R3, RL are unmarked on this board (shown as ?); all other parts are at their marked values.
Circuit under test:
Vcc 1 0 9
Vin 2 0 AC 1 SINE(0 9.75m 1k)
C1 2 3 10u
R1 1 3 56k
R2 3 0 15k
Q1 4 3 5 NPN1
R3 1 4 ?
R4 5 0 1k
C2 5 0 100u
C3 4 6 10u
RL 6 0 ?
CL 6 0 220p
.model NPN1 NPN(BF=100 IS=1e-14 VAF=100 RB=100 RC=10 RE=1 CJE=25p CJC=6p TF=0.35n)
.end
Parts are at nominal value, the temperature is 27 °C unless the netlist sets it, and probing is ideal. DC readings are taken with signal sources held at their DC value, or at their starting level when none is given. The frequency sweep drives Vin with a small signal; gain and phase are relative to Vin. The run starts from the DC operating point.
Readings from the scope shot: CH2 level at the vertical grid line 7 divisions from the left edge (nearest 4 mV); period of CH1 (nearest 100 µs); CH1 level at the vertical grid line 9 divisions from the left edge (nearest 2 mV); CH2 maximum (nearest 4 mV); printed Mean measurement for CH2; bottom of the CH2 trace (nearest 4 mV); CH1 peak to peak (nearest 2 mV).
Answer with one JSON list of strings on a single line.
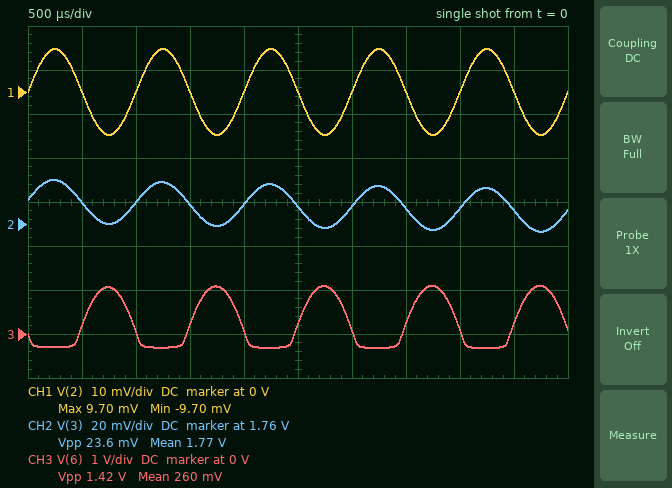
["1.768 V", "1.0 ms", "0 V", "1.780 V", "1.77 V", "1.756 V", "20 mV"]
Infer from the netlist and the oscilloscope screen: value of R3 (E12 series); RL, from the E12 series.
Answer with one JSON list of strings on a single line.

["6.8 kΩ", "5.6 kΩ"]
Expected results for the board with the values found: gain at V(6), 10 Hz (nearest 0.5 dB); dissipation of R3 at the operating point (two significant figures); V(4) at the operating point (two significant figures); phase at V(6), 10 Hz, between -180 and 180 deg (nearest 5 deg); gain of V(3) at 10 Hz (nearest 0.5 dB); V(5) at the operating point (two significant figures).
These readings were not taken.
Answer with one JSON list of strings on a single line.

["24.5 dB", "8.2 mW", "1.5 V", "-90 deg", "-1.0 dB", "1.1 V"]
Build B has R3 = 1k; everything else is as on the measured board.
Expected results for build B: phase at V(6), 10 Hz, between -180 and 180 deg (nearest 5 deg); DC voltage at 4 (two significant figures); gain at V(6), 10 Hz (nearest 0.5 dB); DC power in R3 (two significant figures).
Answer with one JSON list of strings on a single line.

["-85 deg", "7.9 V", "13.0 dB", "1.2 mW"]
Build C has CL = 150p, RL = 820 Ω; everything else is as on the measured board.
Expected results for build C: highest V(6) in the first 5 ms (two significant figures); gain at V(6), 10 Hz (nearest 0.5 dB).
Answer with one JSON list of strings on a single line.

["250 mV", "12.0 dB"]
